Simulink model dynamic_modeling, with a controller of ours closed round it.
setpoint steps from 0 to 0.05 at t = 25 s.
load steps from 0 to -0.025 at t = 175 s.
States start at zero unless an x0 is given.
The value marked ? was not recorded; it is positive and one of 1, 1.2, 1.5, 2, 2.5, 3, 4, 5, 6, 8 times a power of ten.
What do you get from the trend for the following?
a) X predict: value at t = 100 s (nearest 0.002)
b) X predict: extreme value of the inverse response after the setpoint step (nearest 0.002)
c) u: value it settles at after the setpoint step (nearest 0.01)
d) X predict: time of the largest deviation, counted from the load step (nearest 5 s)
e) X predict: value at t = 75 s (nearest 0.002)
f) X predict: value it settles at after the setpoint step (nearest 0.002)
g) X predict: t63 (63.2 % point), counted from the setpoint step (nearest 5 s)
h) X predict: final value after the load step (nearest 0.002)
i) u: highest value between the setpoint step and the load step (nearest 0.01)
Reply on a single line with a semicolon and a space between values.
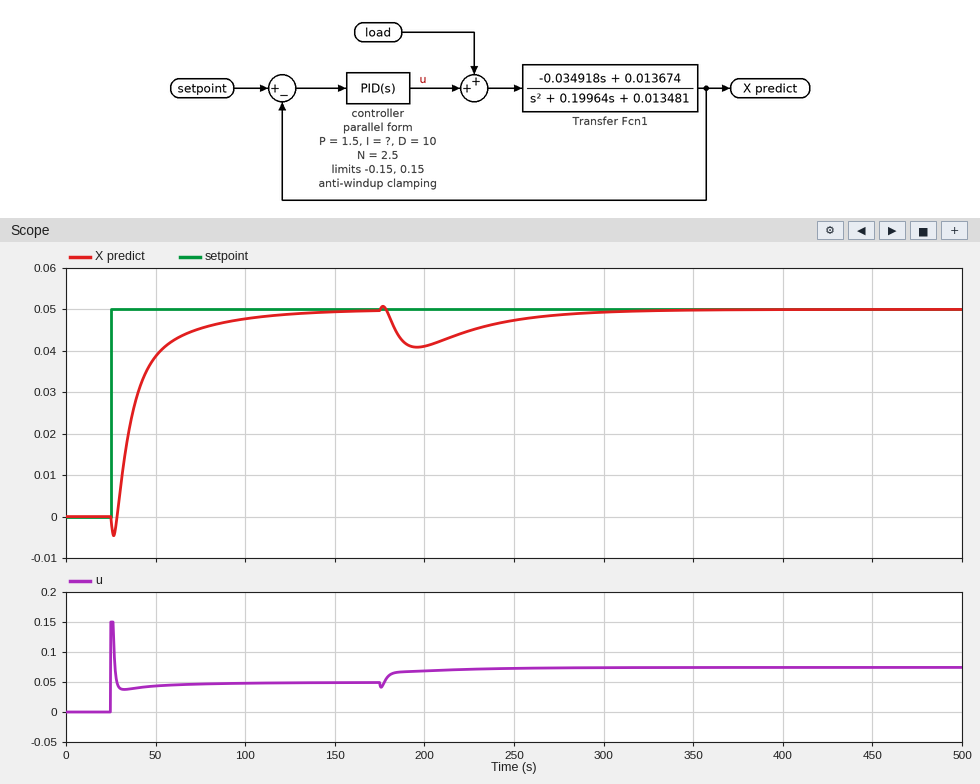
0.048; -0.004; 0.05; 20 s; 0.046; 0.050; 15 s; 0.050; 0.15
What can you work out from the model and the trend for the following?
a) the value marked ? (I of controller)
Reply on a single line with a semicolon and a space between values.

0.05
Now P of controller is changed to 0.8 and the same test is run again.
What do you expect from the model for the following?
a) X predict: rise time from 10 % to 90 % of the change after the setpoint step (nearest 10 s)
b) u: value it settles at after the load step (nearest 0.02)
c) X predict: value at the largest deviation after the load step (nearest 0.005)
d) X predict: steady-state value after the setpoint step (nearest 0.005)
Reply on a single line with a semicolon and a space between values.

40 s; 0.08; 0.040; 0.050
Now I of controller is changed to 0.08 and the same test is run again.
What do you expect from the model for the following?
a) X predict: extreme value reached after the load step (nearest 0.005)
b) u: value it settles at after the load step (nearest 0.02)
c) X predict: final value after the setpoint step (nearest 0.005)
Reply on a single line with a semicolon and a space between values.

0.040; 0.08; 0.050
